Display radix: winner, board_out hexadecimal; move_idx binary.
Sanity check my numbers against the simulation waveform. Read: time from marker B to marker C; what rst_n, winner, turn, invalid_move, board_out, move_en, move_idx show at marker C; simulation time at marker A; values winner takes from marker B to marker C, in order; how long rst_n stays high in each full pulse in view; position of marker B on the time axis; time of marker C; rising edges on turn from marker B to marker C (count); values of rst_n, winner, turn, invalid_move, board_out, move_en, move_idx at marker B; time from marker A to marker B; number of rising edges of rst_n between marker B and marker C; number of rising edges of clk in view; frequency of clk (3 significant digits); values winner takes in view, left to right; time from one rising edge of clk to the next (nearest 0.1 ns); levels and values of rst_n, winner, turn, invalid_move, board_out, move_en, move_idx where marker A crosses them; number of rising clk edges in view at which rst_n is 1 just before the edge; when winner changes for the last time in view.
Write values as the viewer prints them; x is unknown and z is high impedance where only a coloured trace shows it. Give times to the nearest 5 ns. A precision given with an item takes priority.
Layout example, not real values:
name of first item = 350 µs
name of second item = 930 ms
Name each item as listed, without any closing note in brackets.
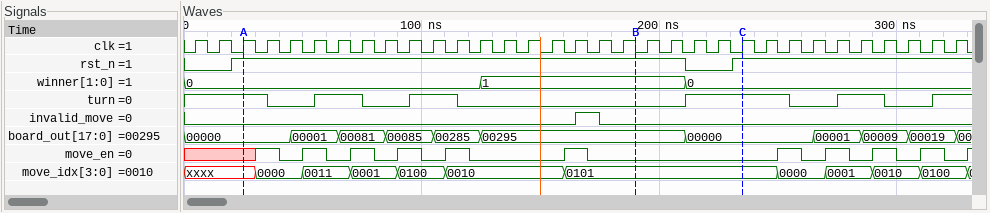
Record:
time from marker B to marker C = 45 ns
what rst_n, winner, turn, invalid_move, board_out, move_en, move_idx show at marker C = rst_n=1, winner=0, turn=1, invalid_move=0, board_out=00000, move_en=0, move_idx=0101
simulation time at marker A = 25 ns
values winner takes from marker B to marker C, in order = 1, 0
how long rst_n stays high in each full pulse in view = 190 ns
position of marker B on the time axis = 190 ns
time of marker C = 235 ns
rising edges on turn from marker B to marker C = 1
values of rst_n, winner, turn, invalid_move, board_out, move_en, move_idx at marker B = rst_n=1, winner=1, turn=0, invalid_move=0, board_out=00295, move_en=0, move_idx=0101
time from marker A to marker B = 165 ns
number of rising edges of rst_n between marker B and marker C = 1
number of rising edges of clk in view = 33
frequency of clk = 100 MHz
values winner takes in view, left to right = 0, 1, 0
time from one rising edge of clk to the next = 10 ns
levels and values of rst_n, winner, turn, invalid_move, board_out, move_en, move_idx where marker A crosses them = rst_n=1, winner=0, turn=1, invalid_move=0, board_out=00000, move_en=x, move_idx=xxxx
number of rising clk edges in view at which rst_n is 1 just before the edge = 29
when winner changes for the last time in view = 210 ns
